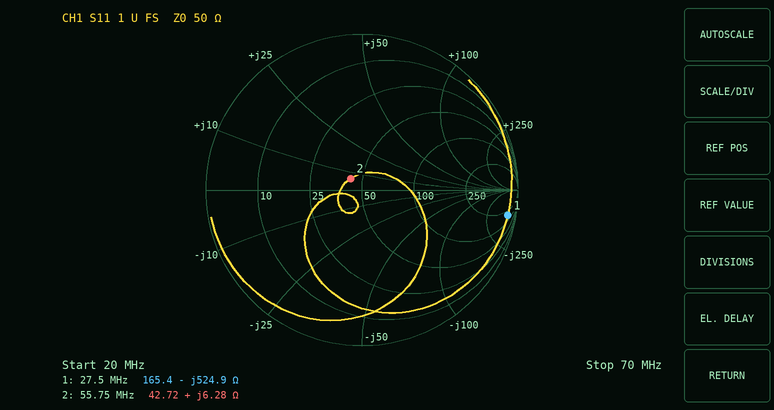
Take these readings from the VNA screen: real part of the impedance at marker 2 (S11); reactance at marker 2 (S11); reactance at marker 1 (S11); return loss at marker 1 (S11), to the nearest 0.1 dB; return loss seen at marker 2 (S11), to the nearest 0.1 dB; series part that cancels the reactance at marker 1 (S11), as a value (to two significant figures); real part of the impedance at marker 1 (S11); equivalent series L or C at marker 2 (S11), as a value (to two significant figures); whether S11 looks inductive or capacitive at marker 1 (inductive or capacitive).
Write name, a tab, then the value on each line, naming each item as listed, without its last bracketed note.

real part of the impedance at marker 2	42.72 Ω
reactance at marker 2	+6.28 Ω
reactance at marker 1	-524.9 Ω
return loss at marker 1 (S11), to the nearest 0.1 dB	0.5 dB
return loss seen at marker 2 (S11), to the nearest 0.1 dB	19.7 dB
series part that cancels the reactance at marker 1 (S11), as a value	3.0 µH
real part of the impedance at marker 1	165.4 Ω
equivalent series L or C at marker 2 (S11), as a value	18 nH
whether S11 looks inductive or capacitive at marker 1	capacitive
